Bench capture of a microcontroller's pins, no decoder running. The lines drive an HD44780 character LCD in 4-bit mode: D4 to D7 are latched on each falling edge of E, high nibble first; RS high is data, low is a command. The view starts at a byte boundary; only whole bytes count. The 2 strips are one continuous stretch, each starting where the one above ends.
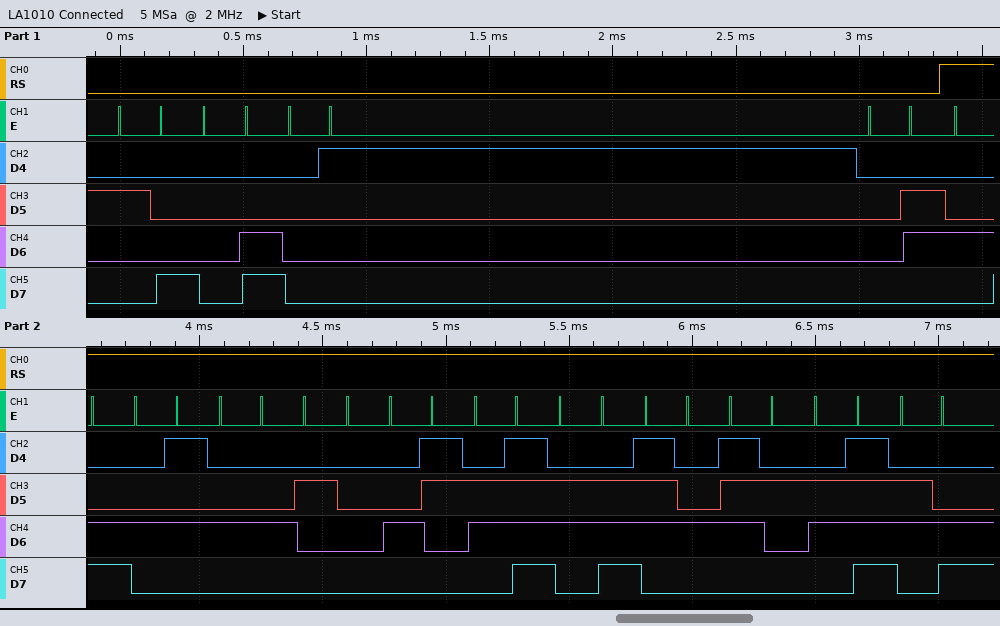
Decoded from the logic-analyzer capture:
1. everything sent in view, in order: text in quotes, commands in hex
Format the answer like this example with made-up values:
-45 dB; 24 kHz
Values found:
0x28 0x0C 0x01 0x06 "LED Control"
